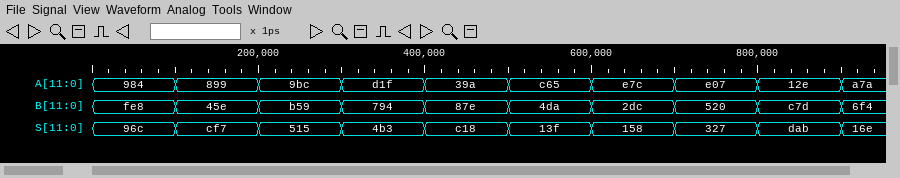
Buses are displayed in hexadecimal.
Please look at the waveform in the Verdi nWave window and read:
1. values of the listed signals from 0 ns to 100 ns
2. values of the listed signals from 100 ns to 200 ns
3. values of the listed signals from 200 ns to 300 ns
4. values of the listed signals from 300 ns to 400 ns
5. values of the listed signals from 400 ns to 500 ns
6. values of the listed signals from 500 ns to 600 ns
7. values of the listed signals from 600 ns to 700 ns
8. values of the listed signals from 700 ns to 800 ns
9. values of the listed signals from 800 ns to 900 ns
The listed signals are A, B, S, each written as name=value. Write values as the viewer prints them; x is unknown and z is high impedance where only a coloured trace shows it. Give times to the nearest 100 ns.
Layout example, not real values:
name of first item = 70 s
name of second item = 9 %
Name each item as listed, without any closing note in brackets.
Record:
values of the listed signals from 0 ns to 100 ns = A=984, B=fe8, S=96c
values of the listed signals from 100 ns to 200 ns = A=899, B=45e, S=cf7
values of the listed signals from 200 ns to 300 ns = A=9bc, B=b59, S=515
values of the listed signals from 300 ns to 400 ns = A=d1f, B=794, S=4b3
values of the listed signals from 400 ns to 500 ns = A=39a, B=87e, S=c18
values of the listed signals from 500 ns to 600 ns = A=c65, B=4da, S=13f
values of the listed signals from 600 ns to 700 ns = A=e7c, B=2dc, S=158
values of the listed signals from 700 ns to 800 ns = A=e07, B=520, S=327
values of the listed signals from 800 ns to 900 ns = A=12e, B=c7d, S=dab
